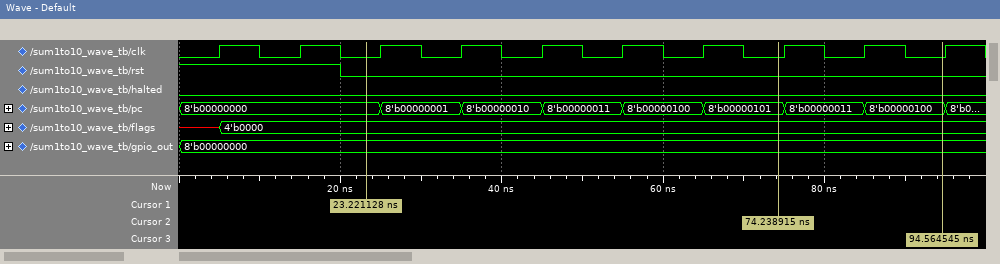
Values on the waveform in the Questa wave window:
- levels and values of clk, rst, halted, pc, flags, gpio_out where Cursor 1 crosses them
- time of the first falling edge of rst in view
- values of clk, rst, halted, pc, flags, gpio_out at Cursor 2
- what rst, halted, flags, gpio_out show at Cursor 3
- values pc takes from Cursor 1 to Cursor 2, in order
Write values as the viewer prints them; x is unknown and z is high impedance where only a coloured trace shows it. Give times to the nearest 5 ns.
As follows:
clk=0, rst=0, halted=0, pc=8'b00000000, flags=4'b0000, gpio_out=8'b00000000
20 ns
clk=0, rst=0, halted=0, pc=8'b00000101, flags=4'b0000, gpio_out=8'b00000000
rst=0, halted=0, flags=4'b0000, gpio_out=8'b00000000
8'b00000000, 8'b00000001, 8'b00000010, 8'b00000011, 8'b00000100, 8'b00000101
